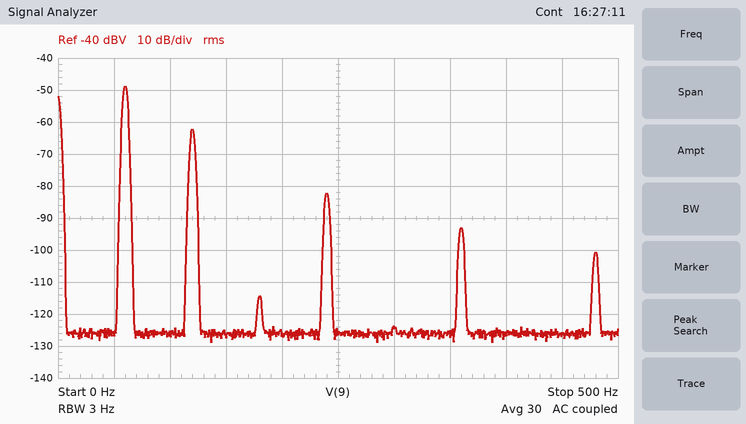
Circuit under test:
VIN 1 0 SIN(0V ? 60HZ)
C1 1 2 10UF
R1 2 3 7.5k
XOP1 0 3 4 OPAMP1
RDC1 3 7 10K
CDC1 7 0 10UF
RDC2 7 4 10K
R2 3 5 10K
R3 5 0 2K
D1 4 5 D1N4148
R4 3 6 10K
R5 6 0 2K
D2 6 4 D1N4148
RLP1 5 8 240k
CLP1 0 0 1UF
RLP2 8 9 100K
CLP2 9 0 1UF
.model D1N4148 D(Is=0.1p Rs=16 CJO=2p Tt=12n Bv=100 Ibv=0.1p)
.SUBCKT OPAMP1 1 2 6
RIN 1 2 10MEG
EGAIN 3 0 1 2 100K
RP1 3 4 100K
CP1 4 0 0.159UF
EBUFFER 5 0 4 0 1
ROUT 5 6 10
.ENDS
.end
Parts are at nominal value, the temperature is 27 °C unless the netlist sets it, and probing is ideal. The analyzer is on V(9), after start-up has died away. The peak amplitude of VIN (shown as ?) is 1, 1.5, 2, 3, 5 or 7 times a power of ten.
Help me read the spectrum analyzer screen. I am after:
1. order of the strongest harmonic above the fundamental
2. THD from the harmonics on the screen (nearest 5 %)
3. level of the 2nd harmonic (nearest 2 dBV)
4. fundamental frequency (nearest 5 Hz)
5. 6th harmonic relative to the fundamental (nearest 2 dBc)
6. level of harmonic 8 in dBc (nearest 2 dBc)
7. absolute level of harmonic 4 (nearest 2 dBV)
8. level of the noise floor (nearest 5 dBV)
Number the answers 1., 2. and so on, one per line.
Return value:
1. 2
2. 20 %
3. -62 dBV
4. 60 Hz
5. -44 dBc
6. -52 dBc
7. -82 dBV
8. -125 dBV
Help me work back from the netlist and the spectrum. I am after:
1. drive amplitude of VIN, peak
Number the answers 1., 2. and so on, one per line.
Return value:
1. 1 V
